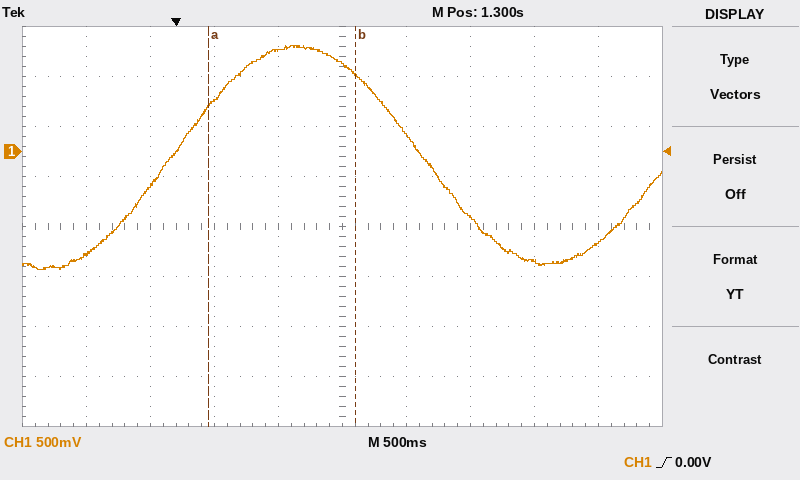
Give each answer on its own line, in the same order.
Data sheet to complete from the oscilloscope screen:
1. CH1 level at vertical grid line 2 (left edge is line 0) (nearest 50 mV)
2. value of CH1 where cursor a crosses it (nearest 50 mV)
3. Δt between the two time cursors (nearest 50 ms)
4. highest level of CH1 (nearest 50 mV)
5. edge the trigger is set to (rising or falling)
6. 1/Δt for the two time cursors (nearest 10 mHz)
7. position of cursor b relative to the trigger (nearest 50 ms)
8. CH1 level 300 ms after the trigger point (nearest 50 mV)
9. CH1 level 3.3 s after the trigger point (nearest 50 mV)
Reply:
-350 mV
450 mV
1.15 s
1.05 V
rising
870 mHz
+1.40 s
500 mV
-900 mV
